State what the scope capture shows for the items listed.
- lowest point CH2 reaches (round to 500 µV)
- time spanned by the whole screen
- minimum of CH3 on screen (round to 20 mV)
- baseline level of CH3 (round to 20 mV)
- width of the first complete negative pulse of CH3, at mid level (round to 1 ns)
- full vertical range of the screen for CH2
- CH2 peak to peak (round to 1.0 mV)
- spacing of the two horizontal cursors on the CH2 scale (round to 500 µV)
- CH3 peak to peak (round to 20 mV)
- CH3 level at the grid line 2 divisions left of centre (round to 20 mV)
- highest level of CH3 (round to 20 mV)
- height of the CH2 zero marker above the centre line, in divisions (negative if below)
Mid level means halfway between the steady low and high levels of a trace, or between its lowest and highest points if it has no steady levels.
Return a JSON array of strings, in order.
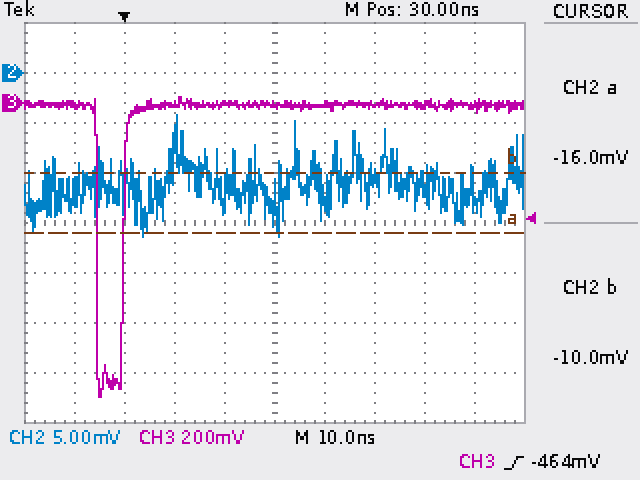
["-16.5 mV", "100 ns", "-1.18 V", "0 mV", "5 ns", "40 mV", "12.0 mV", "6.0 mV", "1.20 V", "0 mV", "20 mV", "+3.0 div"]
